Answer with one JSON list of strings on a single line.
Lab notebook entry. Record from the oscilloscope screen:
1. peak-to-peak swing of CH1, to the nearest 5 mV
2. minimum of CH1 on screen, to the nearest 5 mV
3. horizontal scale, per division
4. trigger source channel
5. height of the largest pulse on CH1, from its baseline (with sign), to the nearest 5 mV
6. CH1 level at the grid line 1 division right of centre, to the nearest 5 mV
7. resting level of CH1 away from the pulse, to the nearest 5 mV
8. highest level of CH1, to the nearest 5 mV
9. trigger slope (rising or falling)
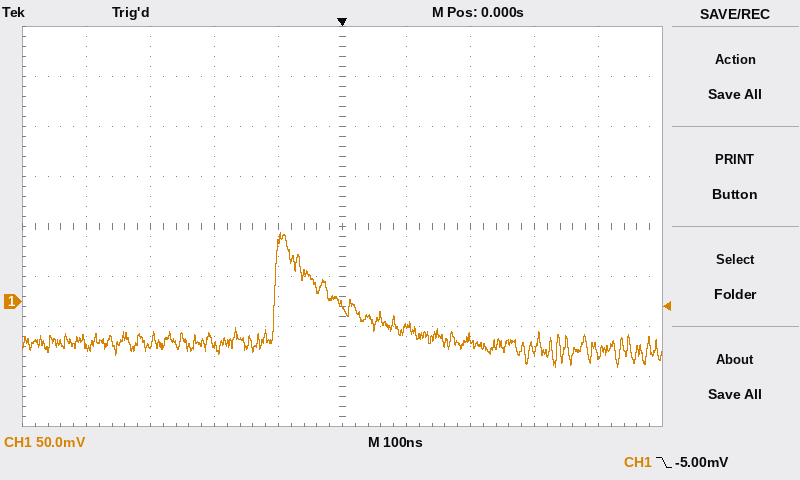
["135 mV", "-65 mV", "100 ns", "CH1", "+110 mV", "-25 mV", "-40 mV", "70 mV", "falling"]
